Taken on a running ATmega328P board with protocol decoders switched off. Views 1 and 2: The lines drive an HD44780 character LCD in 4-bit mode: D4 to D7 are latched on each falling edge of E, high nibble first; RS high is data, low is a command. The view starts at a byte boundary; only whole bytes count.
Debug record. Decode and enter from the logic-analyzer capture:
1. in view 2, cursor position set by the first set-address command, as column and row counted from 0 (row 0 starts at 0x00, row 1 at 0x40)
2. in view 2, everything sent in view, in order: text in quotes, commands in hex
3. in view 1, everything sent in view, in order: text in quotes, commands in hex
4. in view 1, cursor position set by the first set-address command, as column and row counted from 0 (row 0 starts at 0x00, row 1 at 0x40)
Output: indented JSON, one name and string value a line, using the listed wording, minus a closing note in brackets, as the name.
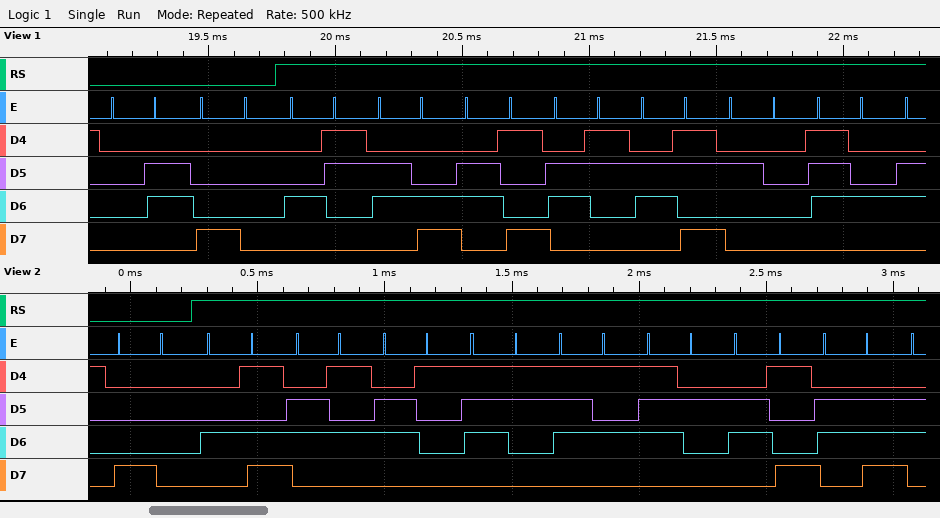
{
  "in view 2, cursor position set by the first set-address command, as column and row counted from 0": "column 0, row 0",
  "in view 2, everything sent in view, in order: text in quotes, commands in hex": "0x80 \"Measurin\"",
  "in view 1, everything sent in view, in order: text in quotes, commands in hex": "0x06 0x80 \"Click t\"",
  "in view 1, cursor position set by the first set-address command, as column and row counted from 0": "column 0, row 0"
}
